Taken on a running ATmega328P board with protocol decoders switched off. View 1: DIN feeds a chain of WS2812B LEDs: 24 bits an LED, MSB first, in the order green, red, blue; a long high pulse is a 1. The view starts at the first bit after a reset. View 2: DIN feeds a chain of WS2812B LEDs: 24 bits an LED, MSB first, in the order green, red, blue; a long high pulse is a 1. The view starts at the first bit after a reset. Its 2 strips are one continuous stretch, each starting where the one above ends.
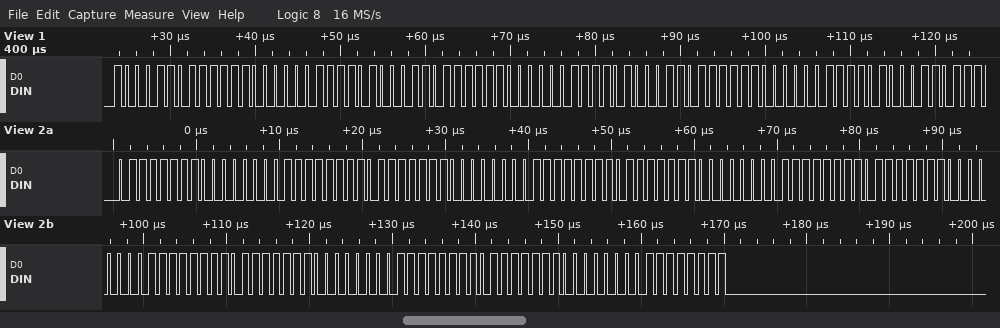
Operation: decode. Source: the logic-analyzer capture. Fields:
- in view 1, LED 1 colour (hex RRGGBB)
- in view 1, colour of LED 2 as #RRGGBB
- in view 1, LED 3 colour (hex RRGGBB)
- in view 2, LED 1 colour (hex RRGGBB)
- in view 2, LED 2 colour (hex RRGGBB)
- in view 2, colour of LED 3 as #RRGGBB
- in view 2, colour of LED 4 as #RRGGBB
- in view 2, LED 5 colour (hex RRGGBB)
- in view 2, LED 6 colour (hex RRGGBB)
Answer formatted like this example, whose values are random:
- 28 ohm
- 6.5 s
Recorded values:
- #F88D1E
- #F88D1E
- #F88D1E
- #007FFF
- #007FFF
- #007FFF
- #007FFF
- #007FFF
- #007FFF
